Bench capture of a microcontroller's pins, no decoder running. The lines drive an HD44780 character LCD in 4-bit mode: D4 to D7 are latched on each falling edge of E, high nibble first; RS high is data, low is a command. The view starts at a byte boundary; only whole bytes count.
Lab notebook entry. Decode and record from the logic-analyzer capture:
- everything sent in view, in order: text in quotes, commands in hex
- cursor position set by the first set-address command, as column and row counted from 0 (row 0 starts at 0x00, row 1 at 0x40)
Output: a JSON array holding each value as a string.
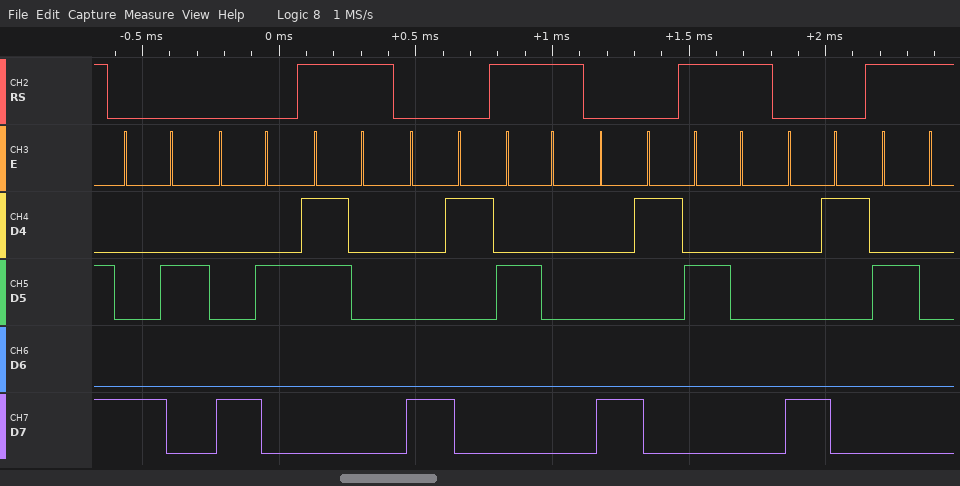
["0x82 0x82 \"0\" 0x81 \" \" 0x81 \" \" 0x81 \" \"", "column 2, row 0"]
